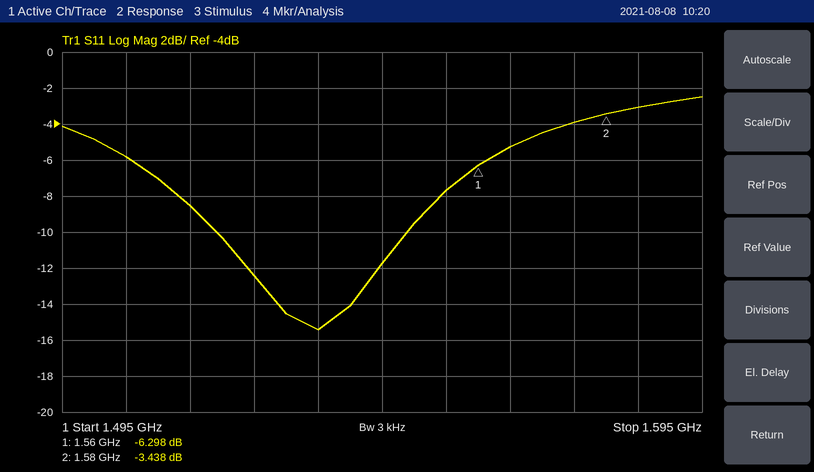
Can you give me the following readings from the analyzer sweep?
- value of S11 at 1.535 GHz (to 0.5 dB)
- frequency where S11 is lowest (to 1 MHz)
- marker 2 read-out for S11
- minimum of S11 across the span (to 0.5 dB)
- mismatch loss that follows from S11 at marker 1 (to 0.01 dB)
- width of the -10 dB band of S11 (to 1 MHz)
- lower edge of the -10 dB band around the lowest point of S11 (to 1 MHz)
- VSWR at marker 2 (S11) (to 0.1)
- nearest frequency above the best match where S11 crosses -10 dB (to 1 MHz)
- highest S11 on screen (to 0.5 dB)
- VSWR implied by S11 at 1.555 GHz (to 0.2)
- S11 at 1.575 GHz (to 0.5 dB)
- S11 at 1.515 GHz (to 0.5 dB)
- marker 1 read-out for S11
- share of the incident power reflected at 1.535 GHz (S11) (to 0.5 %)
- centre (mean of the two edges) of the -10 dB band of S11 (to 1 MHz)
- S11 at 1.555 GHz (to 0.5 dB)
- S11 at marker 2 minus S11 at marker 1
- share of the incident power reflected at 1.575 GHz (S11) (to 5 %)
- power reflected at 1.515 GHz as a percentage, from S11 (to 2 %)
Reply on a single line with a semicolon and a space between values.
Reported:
-15.5 dB; 1.535 GHz; -3.438 dB; -15.5 dB; 1.16 dB; 30 MHz; 1.519 GHz; 5.1; 1.549 GHz; -2.5 dB; 2.4; -4.0 dB; -8.5 dB; -6.298 dB; 3.0 %; 1.534 GHz; -7.5 dB; 2.860 dB; 40 %; 14 %
